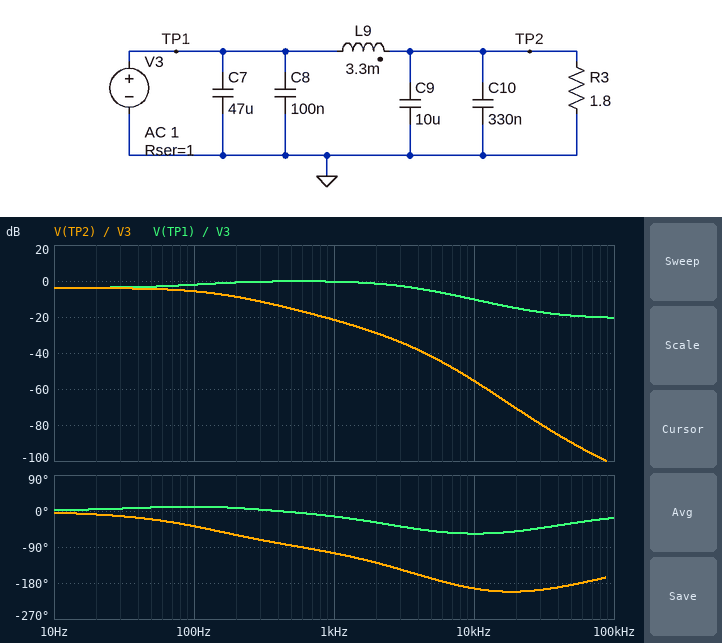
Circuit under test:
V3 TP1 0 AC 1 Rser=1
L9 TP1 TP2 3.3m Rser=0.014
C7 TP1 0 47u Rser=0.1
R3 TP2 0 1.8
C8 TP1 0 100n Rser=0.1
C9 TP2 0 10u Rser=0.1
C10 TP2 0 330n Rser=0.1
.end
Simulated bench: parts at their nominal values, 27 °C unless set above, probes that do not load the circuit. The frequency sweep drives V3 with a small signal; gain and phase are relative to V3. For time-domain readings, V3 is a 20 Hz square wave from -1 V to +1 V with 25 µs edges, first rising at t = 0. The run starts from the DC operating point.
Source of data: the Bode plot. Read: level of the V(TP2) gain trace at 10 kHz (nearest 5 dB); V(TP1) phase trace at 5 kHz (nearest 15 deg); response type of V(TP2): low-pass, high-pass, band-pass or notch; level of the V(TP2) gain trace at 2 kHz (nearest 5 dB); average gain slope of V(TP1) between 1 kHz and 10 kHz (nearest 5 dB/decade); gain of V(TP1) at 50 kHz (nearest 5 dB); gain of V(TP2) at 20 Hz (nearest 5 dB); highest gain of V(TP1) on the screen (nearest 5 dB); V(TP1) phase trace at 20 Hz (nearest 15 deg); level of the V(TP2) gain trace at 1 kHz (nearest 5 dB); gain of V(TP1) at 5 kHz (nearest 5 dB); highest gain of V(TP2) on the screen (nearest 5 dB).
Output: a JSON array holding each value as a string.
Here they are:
["-55 dB", "-45 deg", "low-pass", "-30 dB", "-10 dB/decade", "-20 dB", "-5 dB", "0 dB", "0 deg", "-20 dB", "-5 dB", "-5 dB"]
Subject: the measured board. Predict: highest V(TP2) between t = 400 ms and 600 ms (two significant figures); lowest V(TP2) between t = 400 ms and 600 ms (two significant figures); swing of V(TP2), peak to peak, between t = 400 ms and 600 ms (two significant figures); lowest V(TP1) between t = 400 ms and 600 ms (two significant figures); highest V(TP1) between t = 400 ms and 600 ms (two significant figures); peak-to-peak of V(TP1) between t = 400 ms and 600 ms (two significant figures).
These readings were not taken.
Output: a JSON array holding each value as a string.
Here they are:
["640 mV", "-640 mV", "1.3 V", "-1.3 V", "1.3 V", "2.5 V"]
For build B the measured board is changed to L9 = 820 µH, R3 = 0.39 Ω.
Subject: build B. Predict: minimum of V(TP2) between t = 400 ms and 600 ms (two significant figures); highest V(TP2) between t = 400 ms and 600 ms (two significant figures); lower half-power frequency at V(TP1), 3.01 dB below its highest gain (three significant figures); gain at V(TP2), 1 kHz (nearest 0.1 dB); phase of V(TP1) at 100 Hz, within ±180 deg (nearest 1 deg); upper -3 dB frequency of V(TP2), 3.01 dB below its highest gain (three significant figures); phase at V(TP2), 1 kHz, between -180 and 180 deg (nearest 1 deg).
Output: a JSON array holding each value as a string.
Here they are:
["-280 mV", "280 mV", "225 Hz", "-22.7 dB", "31 deg", "289 Hz", "-93 deg"]
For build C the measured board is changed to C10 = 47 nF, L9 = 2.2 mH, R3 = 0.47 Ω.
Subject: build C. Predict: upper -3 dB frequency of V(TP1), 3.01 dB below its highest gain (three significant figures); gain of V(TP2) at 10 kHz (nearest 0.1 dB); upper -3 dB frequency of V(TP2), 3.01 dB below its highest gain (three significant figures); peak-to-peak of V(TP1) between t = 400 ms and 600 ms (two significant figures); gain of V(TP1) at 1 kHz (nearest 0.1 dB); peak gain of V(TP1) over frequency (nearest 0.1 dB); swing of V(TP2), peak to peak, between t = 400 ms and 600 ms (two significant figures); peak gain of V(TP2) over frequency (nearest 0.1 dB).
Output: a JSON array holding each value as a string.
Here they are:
["3.23 kHz", "-60.1 dB", "110 Hz", "3.1 V", "-0.3 dB", "-0.1 dB", "630 mV", "-10.0 dB"]
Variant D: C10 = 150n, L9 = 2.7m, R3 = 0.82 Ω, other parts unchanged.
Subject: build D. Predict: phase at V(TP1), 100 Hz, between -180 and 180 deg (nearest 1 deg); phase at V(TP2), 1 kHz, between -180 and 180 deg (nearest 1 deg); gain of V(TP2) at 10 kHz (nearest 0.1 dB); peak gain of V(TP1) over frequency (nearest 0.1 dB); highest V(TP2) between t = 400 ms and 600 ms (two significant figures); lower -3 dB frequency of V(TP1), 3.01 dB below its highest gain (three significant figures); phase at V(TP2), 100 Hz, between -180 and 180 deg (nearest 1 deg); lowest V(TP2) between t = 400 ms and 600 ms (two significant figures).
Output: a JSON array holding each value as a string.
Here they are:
["20 deg", "-103 deg", "-57.8 dB", "-0.1 dB", "450 mV", "78.7 Hz", "-44 deg", "-450 mV"]
